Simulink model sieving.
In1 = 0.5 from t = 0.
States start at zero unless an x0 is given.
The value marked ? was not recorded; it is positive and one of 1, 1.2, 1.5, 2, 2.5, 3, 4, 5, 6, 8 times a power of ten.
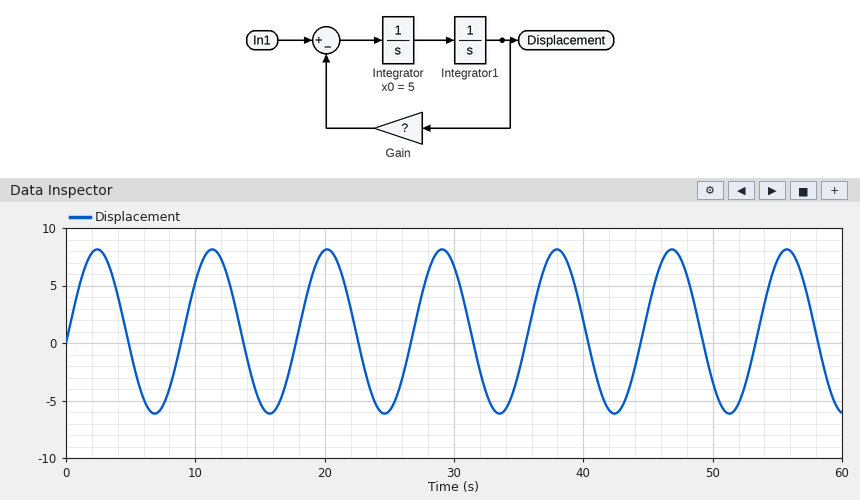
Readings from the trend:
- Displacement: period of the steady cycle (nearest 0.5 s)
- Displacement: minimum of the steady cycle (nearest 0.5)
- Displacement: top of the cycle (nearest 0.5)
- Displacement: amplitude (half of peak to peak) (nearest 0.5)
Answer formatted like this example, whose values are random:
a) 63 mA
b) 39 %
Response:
a) 9.0 s
b) -6.0
c) 8.0
d) 7.0
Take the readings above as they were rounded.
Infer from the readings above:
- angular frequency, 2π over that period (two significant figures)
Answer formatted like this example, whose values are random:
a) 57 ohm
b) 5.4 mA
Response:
a) 0.70 rad/s
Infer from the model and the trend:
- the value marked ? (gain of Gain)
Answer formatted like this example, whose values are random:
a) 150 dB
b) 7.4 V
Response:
a) 0.5
